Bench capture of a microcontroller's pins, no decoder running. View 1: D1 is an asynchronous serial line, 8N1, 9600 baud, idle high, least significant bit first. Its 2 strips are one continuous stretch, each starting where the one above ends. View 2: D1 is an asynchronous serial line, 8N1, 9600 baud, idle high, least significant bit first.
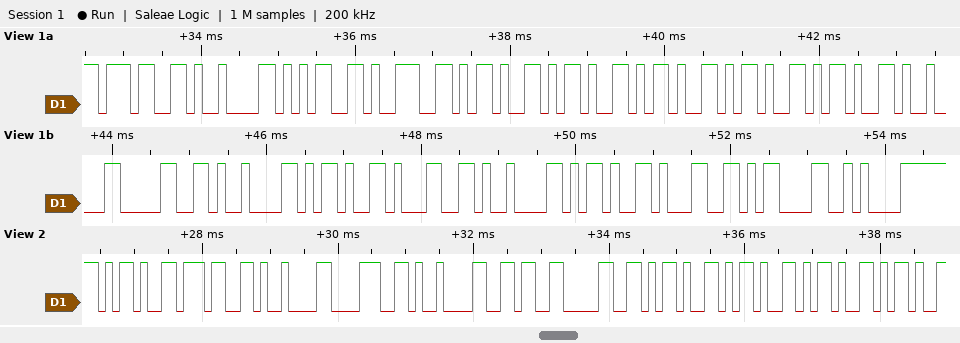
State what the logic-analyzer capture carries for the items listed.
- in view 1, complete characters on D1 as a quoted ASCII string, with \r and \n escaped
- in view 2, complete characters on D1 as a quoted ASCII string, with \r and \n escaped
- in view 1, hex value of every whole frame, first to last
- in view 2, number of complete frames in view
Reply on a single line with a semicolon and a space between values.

"7\t59-----\t0\t-1\t-1\r\n"; "-7\t8\t60----"; 0x37 0x09 0x35 0x39 0x2D 0x2D 0x2D 0x2D 0x2D 0x09 0x30 0x09 0x2D 0x31 0x09 0x2D 0x31 0x0D 0x0A; 11
